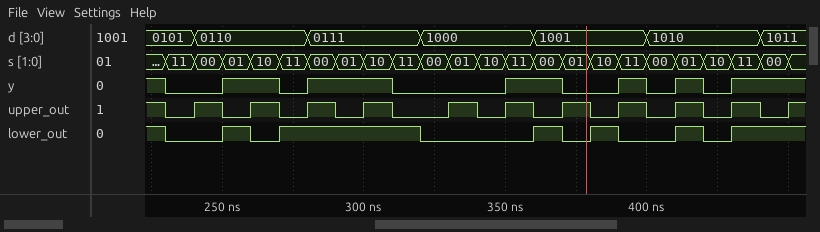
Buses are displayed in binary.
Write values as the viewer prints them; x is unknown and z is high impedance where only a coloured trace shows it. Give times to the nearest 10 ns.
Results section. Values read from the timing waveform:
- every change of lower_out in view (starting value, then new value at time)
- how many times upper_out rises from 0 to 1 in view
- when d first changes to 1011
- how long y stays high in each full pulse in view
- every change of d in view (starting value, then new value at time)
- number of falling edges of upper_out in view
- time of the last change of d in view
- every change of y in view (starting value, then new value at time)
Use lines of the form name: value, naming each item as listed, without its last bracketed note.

every change of lower_out in view: 1, 0 at 230 ns, 1 at 250 ns, 0 at 260 ns, 1 at 270 ns, 0 at 320 ns, 1 at 360 ns, 0 at 370 ns, 1 at 380 ns, 0 at 390 ns, 1 at 410 ns, 0 at 420 ns, 1 at 430 ns
how many times upper_out rises from 0 to 1 in view: 11
when d first changes to 1011: 440 ns
how long y stays high in each full pulse in view: 20 ns, 30 ns, 20 ns, 10 ns, 10 ns
every change of d in view: 0101, 0110 at 240 ns, 0111 at 280 ns, 1000 at 320 ns, 1001 at 360 ns, 1010 at 400 ns, 1011 at 440 ns
number of falling edges of upper_out in view: 11
time of the last change of d in view: 440 ns
every change of y in view: 1, 0 at 230 ns, 1 at 250 ns, 0 at 270 ns, 1 at 280 ns, 0 at 310 ns, 1 at 350 ns, 0 at 370 ns, 1 at 390 ns, 0 at 400 ns, 1 at 410 ns, 0 at 420 ns, 1 at 430 ns
